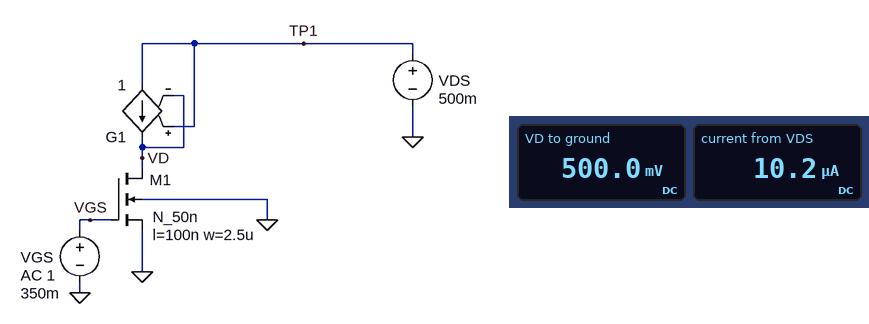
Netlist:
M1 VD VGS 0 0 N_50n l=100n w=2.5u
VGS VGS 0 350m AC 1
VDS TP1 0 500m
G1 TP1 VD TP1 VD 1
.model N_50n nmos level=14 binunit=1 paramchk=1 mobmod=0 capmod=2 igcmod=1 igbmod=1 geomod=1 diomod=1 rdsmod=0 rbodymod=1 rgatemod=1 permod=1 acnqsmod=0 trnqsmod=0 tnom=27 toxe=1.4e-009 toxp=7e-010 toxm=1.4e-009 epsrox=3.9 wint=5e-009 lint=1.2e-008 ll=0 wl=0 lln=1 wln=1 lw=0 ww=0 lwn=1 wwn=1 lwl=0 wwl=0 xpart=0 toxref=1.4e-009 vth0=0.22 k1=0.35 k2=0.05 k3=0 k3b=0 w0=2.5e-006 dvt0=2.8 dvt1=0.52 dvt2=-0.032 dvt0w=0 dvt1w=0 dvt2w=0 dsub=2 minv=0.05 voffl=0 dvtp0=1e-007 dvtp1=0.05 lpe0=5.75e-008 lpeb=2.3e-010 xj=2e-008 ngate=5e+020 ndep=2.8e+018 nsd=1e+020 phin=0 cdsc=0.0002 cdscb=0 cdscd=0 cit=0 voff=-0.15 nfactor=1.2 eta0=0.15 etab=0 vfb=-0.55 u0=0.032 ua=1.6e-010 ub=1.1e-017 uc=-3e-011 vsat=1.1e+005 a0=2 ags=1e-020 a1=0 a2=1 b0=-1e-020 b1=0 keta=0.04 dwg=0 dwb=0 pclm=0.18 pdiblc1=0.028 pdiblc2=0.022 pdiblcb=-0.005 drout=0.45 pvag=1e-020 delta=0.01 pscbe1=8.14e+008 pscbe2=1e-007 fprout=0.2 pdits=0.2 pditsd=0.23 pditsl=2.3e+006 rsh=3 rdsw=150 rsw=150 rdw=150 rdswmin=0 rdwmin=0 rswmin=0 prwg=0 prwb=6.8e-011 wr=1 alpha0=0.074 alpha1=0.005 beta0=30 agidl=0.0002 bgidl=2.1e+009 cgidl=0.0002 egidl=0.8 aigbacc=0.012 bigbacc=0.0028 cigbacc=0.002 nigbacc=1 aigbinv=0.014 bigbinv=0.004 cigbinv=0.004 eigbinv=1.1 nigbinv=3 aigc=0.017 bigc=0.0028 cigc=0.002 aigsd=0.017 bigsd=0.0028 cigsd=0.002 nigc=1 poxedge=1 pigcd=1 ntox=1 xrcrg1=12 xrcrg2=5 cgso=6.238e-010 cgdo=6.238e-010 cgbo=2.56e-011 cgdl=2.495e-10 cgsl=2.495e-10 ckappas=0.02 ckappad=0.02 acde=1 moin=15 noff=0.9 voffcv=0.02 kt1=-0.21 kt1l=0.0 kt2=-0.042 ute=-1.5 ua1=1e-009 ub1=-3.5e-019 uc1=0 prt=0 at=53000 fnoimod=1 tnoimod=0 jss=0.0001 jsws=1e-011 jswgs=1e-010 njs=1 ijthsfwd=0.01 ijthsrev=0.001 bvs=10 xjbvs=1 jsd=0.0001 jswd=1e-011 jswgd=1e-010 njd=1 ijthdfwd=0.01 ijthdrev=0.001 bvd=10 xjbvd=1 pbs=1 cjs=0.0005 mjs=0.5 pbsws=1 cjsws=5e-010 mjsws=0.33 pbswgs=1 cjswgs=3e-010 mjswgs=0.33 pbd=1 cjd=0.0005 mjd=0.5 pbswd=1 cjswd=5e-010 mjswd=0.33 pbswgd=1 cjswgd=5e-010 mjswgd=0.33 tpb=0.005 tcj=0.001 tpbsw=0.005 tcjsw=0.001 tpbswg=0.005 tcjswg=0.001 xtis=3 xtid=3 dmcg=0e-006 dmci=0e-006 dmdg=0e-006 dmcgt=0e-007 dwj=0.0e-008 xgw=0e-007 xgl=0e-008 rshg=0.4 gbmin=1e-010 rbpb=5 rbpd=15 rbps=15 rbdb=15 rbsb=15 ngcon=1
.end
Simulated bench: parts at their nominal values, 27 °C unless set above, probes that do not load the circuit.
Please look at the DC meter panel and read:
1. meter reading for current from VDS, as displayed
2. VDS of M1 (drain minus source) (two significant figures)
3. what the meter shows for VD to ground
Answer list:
10.2 µA
500 mV
500.0 mV
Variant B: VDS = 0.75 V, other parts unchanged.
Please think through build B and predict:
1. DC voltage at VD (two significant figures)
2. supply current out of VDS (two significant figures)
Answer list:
750 mV
12 µA
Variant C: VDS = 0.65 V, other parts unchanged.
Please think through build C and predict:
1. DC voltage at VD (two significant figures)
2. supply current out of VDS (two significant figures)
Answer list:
650 mV
11 µA
